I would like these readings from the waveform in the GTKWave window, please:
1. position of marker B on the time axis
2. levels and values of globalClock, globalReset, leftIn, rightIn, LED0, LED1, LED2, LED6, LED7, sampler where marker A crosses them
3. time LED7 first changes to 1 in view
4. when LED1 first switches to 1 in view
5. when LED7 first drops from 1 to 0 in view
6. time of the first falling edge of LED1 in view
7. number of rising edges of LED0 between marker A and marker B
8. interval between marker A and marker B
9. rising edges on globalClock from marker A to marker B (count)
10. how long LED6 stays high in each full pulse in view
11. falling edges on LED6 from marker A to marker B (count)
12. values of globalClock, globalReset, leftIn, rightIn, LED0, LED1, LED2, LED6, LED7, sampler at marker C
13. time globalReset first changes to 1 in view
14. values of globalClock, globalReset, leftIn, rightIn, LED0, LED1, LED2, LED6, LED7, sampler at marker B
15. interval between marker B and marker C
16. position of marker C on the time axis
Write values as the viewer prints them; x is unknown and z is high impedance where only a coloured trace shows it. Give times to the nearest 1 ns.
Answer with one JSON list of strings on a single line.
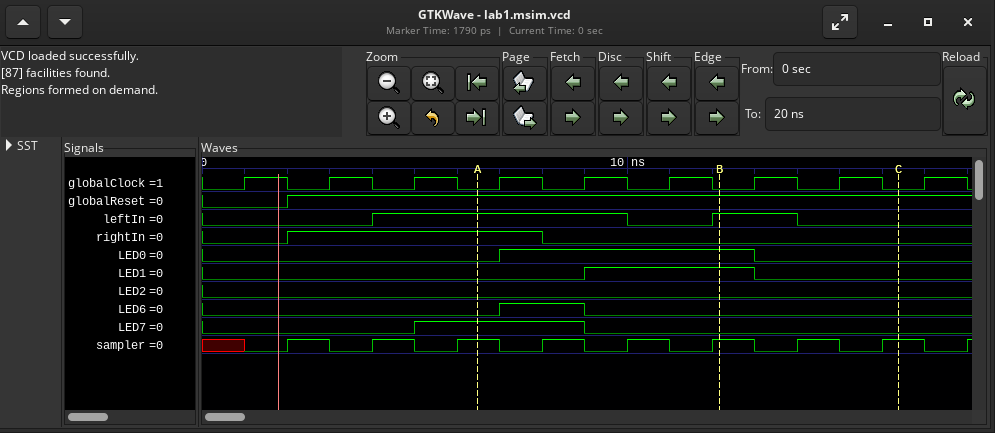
["12 ns", "globalClock=0, globalReset=1, leftIn=1, rightIn=1, LED0=0, LED1=0, LED2=0, LED6=0, LED7=1, sampler=1", "5 ns", "9 ns", "9 ns", "13 ns", "1", "6 ns", "3", "2 ns", "1", "globalClock=0, globalReset=1, leftIn=0, rightIn=0, LED0=0, LED1=0, LED2=0, LED6=0, LED7=0, sampler=1", "2 ns", "globalClock=0, globalReset=1, leftIn=1, rightIn=0, LED0=1, LED1=1, LED2=0, LED6=0, LED7=0, sampler=1", "4 ns", "16 ns"]
